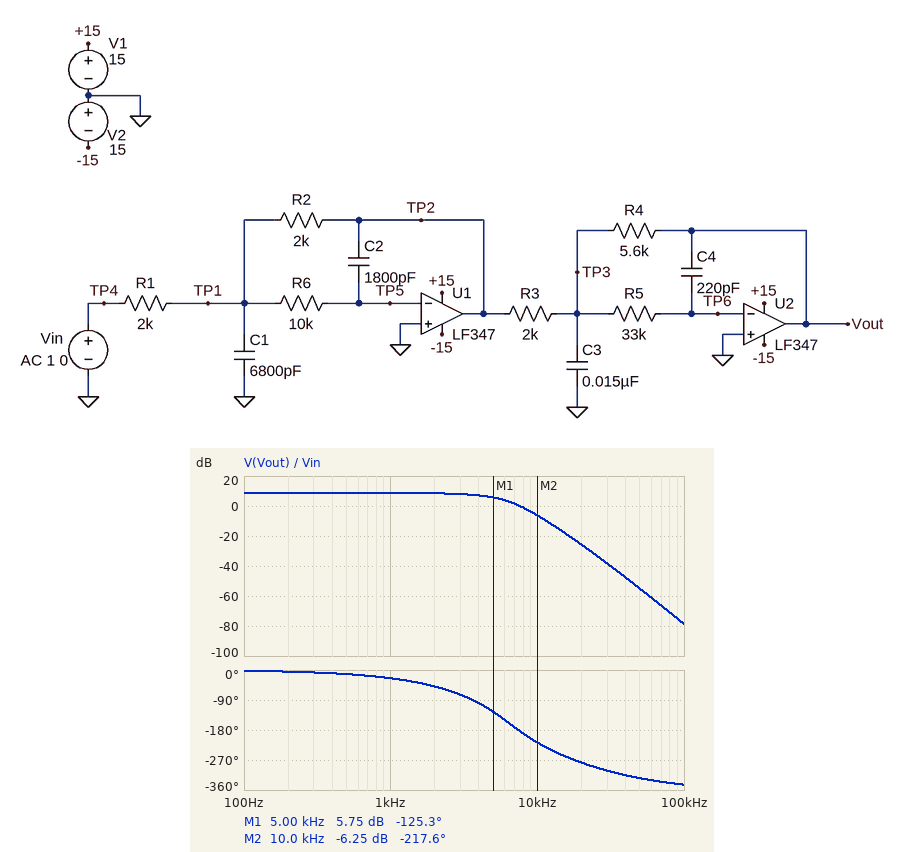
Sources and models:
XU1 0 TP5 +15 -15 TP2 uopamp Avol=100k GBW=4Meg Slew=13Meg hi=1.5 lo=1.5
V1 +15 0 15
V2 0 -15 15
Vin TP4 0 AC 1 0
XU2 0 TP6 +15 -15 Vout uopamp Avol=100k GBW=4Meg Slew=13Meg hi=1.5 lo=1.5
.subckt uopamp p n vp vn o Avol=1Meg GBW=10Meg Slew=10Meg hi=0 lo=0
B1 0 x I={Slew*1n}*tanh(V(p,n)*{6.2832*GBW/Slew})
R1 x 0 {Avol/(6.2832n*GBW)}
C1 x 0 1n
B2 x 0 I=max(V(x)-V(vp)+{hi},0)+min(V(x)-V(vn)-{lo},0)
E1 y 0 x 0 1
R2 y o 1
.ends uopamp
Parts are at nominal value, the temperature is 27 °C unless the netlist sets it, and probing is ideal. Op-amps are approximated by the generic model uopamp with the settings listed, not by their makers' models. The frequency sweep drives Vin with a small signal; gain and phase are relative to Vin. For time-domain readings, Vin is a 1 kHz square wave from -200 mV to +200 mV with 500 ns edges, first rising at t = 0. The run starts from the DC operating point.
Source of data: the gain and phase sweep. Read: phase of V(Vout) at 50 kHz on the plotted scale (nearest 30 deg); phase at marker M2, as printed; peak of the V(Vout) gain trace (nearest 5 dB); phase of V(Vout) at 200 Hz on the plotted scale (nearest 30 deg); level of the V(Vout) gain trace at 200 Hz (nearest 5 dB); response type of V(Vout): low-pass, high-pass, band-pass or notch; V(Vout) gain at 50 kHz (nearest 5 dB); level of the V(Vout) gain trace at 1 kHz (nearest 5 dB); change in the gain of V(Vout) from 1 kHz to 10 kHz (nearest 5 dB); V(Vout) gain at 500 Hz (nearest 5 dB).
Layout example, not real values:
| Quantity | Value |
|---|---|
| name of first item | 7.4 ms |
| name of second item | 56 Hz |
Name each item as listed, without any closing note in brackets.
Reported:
| Quantity | Value |
|---|---|
| phase of V(Vout) at 50 kHz on the plotted scale | -330 deg |
| phase at marker M2, as printed | -217.6 deg |
| peak of the V(Vout) gain trace | 10 dB |
| phase of V(Vout) at 200 Hz on the plotted scale | 0 deg |
| level of the V(Vout) gain trace at 200 Hz | 10 dB |
| response type of V(Vout): low-pass, high-pass, band-pass or notch | low-pass |
| V(Vout) gain at 50 kHz | -55 dB |
| level of the V(Vout) gain trace at 1 kHz | 10 dB |
| change in the gain of V(Vout) from 1 kHz to 10 kHz | -15 dB |
| V(Vout) gain at 500 Hz | 10 dB |
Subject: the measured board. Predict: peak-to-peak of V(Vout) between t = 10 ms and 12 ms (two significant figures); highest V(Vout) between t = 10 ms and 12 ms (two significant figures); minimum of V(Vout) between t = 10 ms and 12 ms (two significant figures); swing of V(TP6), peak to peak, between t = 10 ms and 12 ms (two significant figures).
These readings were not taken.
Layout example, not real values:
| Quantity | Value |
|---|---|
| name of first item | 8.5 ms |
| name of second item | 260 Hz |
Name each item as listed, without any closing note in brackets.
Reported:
| Quantity | Value |
|---|---|
| peak-to-peak of V(Vout) between t = 10 ms and 12 ms | 1.2 V |
| highest V(Vout) between t = 10 ms and 12 ms | 580 mV |
| minimum of V(Vout) between t = 10 ms and 12 ms | -580 mV |
| swing of V(TP6), peak to peak, between t = 10 ms and 12 ms | 1.2 mV |
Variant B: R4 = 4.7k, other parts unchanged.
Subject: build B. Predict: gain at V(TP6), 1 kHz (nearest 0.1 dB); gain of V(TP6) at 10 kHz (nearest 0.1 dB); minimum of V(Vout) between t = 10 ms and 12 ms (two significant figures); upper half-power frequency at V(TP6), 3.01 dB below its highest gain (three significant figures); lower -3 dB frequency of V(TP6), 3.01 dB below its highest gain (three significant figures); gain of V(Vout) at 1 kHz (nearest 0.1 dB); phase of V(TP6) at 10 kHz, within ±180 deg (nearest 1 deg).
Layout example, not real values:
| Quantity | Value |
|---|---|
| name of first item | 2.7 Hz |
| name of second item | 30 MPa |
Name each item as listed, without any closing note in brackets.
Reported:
| Quantity | Value |
|---|---|
| gain at V(TP6), 1 kHz | -64.7 dB |
| gain of V(TP6) at 10 kHz | -58.1 dB |
| minimum of V(Vout) between t = 10 ms and 12 ms | -480 mV |
| upper half-power frequency at V(TP6), 3.01 dB below its highest gain | 8.79 kHz |
| lower -3 dB frequency of V(TP6), 3.01 dB below its highest gain | 2.92 kHz |
| gain of V(Vout) at 1 kHz | 7.3 dB |
| phase of V(TP6) at 10 kHz, within ±180 deg | 57 deg |
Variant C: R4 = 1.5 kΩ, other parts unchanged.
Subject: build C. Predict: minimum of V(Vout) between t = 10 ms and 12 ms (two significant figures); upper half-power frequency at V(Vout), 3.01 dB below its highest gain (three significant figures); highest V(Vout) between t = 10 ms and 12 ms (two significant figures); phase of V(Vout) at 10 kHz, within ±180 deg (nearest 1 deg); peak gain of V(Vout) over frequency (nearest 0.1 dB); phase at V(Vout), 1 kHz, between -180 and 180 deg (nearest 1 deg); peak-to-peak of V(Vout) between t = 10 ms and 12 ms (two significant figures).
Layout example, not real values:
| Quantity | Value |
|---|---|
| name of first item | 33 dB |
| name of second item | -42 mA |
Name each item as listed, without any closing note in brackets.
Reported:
| Quantity | Value |
|---|---|
| minimum of V(Vout) between t = 10 ms and 12 ms | -150 mV |
| upper half-power frequency at V(Vout), 3.01 dB below its highest gain | 5.44 kHz |
| highest V(Vout) between t = 10 ms and 12 ms | 150 mV |
| phase of V(Vout) at 10 kHz, within ±180 deg | -156 deg |
| peak gain of V(Vout) over frequency | -2.5 dB |
| phase at V(Vout), 1 kHz, between -180 and 180 deg | -19 deg |
| peak-to-peak of V(Vout) between t = 10 ms and 12 ms | 300 mV |
